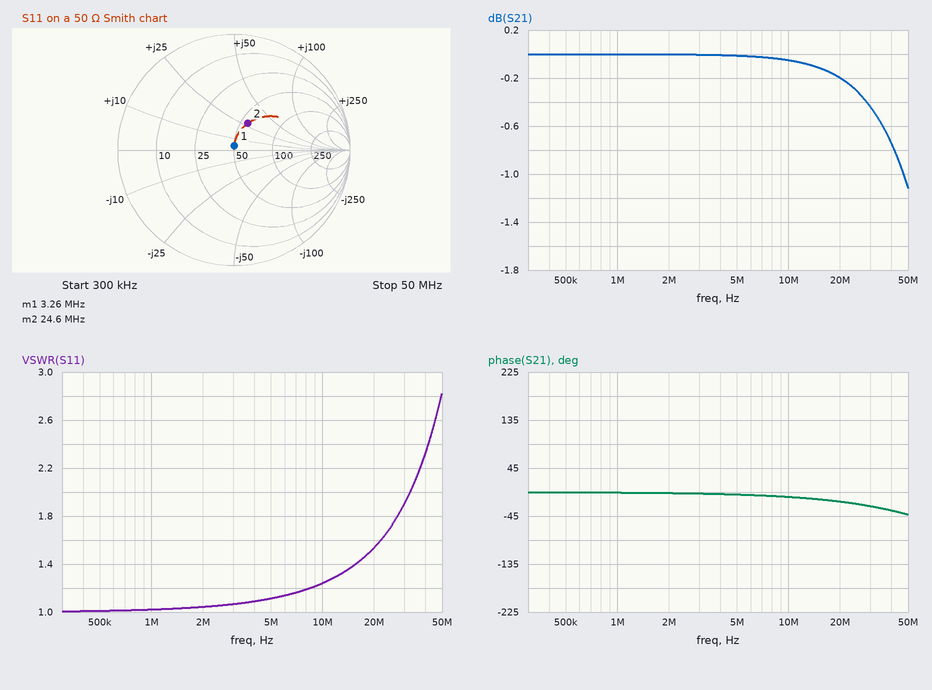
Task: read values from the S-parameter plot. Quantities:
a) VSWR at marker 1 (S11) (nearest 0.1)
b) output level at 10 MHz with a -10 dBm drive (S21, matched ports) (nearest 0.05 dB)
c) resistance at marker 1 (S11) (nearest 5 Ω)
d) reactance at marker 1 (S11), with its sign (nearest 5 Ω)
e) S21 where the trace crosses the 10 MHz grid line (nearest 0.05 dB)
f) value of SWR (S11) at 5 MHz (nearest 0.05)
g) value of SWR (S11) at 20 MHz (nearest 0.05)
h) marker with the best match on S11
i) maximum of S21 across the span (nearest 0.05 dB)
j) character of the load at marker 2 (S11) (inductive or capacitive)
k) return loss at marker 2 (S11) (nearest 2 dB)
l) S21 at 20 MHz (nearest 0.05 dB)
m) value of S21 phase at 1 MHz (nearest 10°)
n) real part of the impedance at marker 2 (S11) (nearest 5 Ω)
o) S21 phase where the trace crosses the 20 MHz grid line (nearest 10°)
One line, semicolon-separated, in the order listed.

1.1; -10.05 dBm; 50 Ω; +5 Ω; -0.05 dB; 1.10; 1.55; marker 1; 0.00 dB; inductive; 12 dB; -0.20 dB; 0°; 55 Ω; -20°
